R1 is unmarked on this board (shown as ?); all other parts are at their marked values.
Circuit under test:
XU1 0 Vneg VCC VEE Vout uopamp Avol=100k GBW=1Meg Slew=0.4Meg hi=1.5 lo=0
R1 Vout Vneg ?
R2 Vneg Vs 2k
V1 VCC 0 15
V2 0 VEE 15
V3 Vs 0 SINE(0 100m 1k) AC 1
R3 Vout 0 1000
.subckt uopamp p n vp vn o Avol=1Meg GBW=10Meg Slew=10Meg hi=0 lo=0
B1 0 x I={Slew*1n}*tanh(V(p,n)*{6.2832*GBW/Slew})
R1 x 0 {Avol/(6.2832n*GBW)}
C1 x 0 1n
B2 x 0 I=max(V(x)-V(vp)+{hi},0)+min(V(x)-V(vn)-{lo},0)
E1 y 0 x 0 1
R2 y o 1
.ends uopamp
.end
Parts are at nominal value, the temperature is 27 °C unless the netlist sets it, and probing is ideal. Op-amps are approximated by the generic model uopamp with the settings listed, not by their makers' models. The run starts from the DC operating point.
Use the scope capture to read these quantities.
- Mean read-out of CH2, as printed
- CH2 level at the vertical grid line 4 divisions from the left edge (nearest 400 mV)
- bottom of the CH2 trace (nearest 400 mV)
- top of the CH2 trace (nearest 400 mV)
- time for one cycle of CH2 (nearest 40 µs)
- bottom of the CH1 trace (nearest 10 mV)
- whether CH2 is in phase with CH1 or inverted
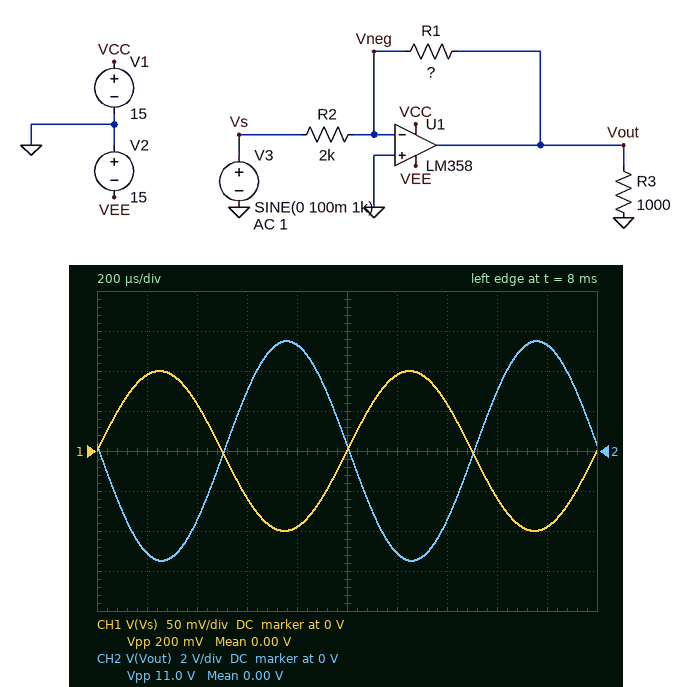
0.00 V
5.2 V
-5.6 V
5.6 V
1.00 ms
-100 mV
inverted
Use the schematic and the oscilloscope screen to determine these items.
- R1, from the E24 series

110 kΩ
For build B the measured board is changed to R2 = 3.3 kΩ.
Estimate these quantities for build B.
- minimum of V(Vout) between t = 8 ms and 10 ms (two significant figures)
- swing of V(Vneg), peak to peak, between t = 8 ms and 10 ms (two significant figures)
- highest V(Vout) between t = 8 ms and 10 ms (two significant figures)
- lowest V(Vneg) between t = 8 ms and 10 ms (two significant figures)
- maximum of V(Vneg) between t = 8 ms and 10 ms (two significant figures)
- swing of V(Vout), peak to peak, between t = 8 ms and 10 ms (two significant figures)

-3.3 V
6.7 mV
3.3 V
-3.3 mV
3.3 mV
6.7 V
